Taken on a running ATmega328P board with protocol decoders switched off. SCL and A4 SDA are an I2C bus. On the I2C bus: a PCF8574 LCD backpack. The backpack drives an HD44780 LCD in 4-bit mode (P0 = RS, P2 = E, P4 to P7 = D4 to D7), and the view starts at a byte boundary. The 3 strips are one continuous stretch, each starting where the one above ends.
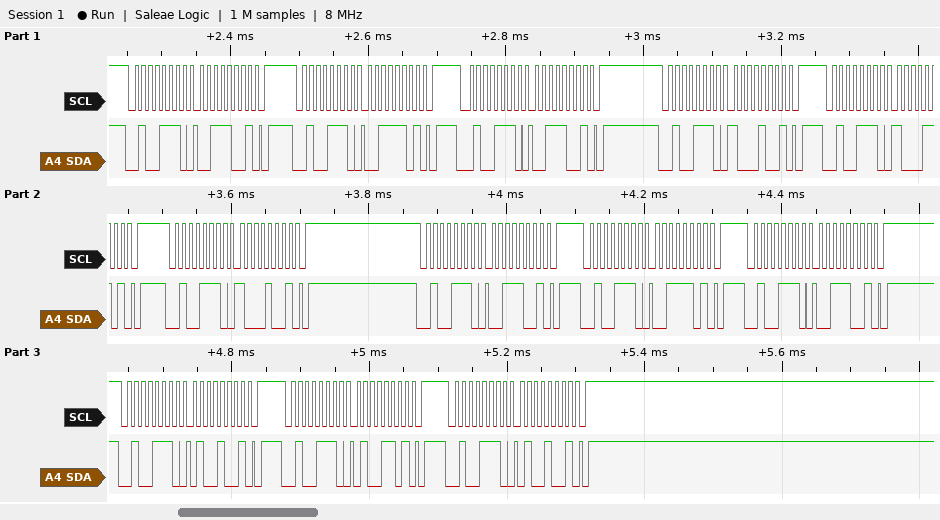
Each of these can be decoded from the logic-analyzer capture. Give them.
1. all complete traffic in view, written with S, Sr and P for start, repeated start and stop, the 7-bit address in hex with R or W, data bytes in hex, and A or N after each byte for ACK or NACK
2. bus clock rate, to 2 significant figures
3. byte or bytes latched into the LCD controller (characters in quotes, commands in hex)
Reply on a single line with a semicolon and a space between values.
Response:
S 27W A 39 A P S 27W A 3D A P S 27W A 39 A P S 27W A 89 A P S 27W A 8D A P S 27W A 89 A P S 27W A 39 A P S 27W A 3D A P S 27W A 39 A P S 27W A 49 A P S 27W A 4D A P S 27W A 49 A P; 100 kHz; '8' '4'
